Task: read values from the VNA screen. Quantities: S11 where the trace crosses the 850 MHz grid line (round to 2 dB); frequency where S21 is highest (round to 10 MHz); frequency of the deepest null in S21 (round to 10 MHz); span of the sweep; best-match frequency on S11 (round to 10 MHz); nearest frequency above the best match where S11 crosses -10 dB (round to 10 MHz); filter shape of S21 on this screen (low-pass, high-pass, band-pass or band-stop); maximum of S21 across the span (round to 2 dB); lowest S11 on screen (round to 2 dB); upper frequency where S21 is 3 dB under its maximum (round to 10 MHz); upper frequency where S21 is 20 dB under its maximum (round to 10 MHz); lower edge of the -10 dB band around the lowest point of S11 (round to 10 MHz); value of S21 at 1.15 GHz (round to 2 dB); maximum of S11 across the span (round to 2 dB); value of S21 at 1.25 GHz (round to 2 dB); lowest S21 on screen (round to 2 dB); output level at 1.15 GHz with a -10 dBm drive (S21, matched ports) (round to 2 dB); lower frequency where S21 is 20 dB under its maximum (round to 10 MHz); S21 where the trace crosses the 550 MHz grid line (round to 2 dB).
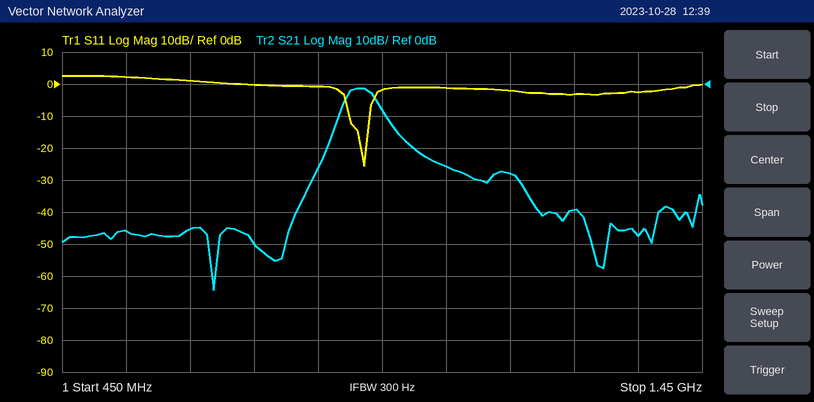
0 dB
910 MHz
690 MHz
1 GHz
920 MHz
930 MHz
band-pass
-2 dB
-26 dB
940 MHz
1.01 GHz
900 MHz
-28 dB
2 dB
-40 dB
-64 dB
-38 dBm
860 MHz
-46 dB
